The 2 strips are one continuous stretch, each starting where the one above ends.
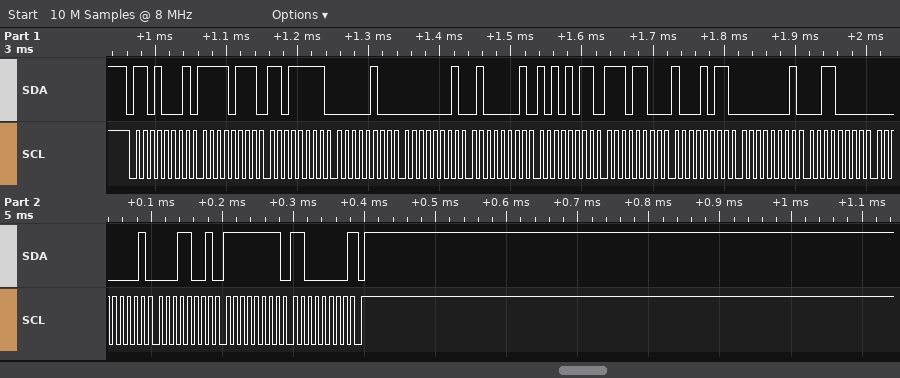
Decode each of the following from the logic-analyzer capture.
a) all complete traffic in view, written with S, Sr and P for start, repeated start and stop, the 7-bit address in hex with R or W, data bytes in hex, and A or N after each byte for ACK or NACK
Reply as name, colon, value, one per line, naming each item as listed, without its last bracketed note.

all complete traffic in view, written with S, Sr and P for start, repeated start and stop, the 7-bit address in hex with R or W, data bytes in hex, and A or N after each byte for ACK or NACK: S 68R A F7 A DF A 04 A 01 A 41 A AB A EC A 8B A 01 A 30 A 01 A 19 A FF A C0 N P
